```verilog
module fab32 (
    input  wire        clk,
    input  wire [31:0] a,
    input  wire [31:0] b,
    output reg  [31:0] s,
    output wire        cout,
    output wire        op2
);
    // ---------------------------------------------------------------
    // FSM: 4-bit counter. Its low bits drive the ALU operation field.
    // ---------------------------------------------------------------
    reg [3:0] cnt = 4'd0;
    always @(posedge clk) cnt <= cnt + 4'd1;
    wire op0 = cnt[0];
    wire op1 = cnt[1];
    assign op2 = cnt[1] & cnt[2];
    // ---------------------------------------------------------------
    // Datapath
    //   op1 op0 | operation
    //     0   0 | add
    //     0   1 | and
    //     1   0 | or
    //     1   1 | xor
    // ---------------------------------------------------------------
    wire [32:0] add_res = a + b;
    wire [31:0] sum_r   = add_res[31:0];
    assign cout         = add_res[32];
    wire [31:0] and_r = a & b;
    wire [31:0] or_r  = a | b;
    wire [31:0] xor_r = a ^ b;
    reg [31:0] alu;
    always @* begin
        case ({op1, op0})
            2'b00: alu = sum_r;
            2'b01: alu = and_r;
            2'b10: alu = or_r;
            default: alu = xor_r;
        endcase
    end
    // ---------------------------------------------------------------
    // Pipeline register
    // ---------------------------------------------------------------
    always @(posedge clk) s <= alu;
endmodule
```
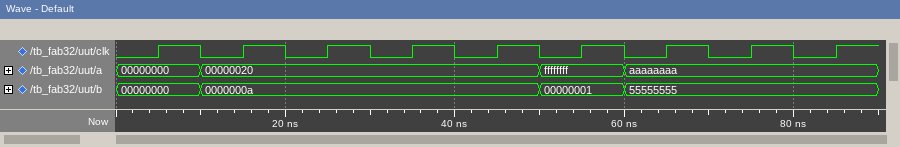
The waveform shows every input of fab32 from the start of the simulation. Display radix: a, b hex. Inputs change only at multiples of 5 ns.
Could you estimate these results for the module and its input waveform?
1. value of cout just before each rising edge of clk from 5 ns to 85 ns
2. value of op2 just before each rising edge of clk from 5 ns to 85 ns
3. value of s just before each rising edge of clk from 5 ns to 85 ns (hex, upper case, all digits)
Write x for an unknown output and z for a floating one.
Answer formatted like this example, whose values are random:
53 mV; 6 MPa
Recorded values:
0 0 0 0 0 1 0 0 0; 0 0 0 0 0 0 1 1 0; x, 00000000, 00000000, 0000002A, 0000002A, 0000002A, 00000001, FFFFFFFF, FFFFFFFF
